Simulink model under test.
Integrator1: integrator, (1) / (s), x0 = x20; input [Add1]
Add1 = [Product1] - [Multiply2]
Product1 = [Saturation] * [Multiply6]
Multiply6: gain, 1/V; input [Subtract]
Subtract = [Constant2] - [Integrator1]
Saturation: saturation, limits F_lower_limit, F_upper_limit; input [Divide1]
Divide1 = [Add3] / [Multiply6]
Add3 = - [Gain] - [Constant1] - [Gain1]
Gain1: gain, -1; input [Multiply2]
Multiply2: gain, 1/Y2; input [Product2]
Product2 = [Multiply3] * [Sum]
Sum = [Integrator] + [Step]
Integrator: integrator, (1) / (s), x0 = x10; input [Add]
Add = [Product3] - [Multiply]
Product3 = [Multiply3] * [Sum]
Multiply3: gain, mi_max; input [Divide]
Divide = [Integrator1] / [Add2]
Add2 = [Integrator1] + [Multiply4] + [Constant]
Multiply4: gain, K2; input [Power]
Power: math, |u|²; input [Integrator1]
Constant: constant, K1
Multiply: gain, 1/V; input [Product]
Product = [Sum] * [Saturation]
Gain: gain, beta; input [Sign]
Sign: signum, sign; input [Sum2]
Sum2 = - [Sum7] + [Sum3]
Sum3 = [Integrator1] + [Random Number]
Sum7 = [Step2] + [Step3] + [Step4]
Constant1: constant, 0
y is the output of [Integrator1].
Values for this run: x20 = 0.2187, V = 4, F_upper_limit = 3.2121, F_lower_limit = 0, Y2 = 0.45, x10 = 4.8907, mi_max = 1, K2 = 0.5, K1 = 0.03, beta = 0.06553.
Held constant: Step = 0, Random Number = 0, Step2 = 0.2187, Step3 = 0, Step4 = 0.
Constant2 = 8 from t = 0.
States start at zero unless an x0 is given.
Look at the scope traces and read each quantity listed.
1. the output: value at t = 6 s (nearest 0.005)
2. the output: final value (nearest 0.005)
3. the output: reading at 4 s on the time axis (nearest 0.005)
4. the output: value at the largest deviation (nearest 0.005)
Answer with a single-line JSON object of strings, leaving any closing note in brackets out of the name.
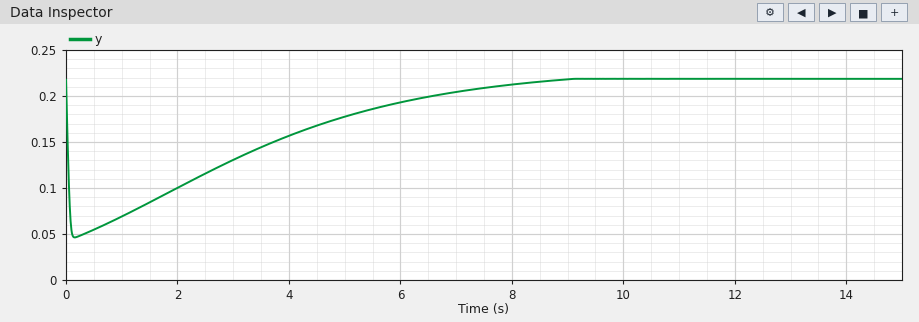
{"the output: value at t = 6 s": "0.195", "the output: final value": "0.220", "the output: reading at 4 s on the time axis": "0.155", "the output: value at the largest deviation": "0.045"}
